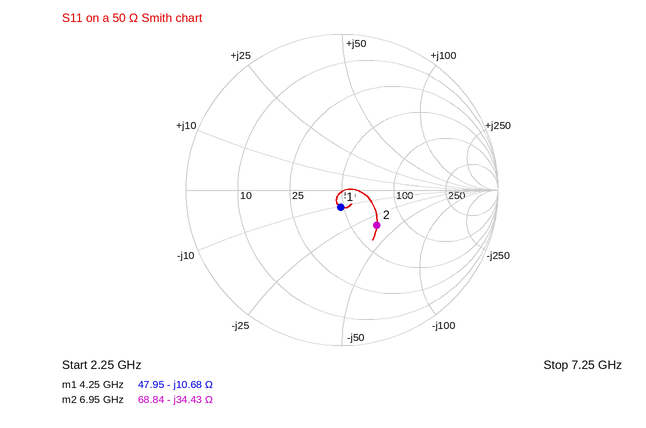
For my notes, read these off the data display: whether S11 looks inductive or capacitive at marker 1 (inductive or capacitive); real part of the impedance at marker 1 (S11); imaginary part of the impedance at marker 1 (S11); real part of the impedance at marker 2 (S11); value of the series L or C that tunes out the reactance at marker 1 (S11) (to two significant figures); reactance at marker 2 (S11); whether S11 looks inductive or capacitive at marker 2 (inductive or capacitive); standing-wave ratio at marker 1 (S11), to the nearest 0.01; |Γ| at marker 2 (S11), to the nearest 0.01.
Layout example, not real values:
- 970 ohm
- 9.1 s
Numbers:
- capacitive
- 47.95 Ω
- -10.68 Ω
- 68.84 Ω
- 400 pH
- -34.43 Ω
- capacitive
- 1.25
- 0.32
